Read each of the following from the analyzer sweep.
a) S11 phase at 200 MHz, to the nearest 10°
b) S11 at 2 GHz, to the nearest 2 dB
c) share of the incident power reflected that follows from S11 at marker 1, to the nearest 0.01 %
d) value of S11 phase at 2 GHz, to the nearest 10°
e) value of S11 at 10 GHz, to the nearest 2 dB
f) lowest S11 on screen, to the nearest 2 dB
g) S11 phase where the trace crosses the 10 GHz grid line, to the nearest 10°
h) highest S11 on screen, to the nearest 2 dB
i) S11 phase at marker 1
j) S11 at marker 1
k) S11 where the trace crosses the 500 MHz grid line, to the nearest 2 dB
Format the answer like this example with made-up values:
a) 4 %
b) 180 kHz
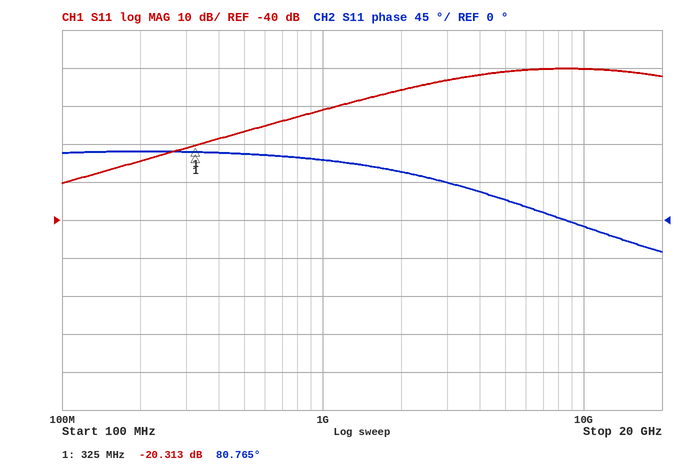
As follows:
a) 80°
b) -6 dB
c) 0.93 %
d) 60°
e) 0 dB
f) -30 dB
g) -10°
h) 0 dB
i) 80.765°
j) -20.313 dB
k) -16 dB
